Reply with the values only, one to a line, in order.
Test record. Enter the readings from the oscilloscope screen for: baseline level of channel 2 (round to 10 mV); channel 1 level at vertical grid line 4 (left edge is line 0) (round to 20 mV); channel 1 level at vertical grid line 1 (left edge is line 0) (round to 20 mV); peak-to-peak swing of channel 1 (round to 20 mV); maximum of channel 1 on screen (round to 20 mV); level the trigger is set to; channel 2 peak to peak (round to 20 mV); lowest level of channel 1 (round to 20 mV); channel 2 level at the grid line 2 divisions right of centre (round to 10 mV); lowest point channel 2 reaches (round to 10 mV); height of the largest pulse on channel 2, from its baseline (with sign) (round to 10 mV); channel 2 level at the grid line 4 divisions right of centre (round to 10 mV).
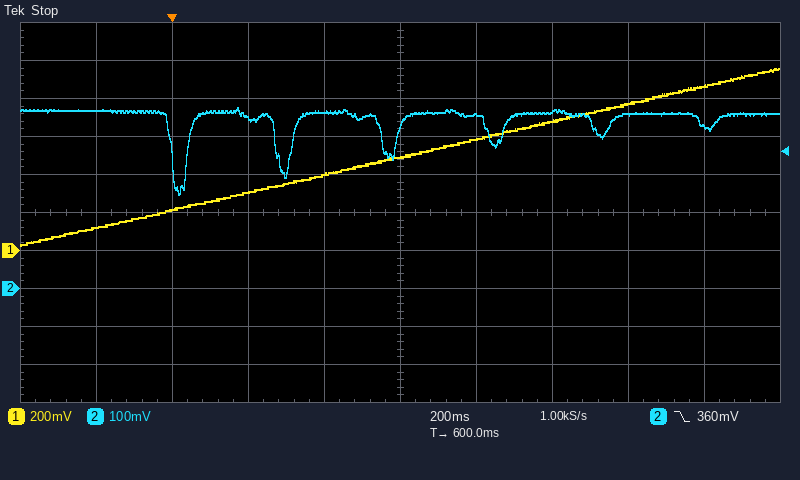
460 mV
400 mV
120 mV
940 mV
960 mV
360 mV
220 mV
20 mV
470 mV
250 mV
-210 mV
430 mV
